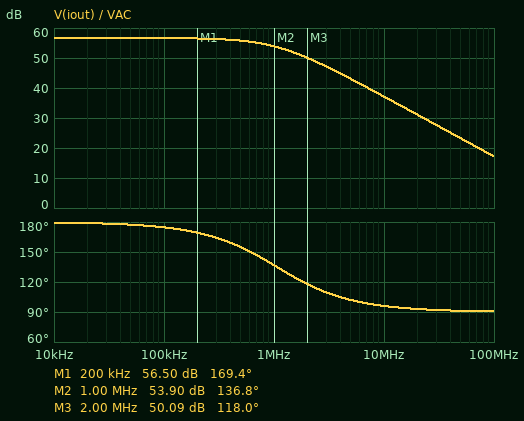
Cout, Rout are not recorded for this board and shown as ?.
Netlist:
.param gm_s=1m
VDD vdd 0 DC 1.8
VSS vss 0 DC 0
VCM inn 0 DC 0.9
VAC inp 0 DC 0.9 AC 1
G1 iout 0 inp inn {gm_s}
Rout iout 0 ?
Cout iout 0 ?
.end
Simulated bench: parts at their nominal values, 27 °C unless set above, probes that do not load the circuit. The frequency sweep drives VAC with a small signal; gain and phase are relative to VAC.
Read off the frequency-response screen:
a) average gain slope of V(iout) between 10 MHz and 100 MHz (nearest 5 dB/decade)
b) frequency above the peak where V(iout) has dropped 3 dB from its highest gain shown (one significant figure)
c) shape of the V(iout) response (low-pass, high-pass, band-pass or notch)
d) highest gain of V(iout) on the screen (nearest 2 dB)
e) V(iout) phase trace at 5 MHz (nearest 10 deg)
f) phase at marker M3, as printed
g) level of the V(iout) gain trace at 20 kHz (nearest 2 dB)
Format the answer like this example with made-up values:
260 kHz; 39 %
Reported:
-20 dB/decade; 1 MHz; low-pass; 56 dB; 100 deg; 118.0 deg; 56 dB
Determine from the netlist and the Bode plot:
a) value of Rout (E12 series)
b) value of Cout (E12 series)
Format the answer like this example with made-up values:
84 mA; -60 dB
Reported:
680 kΩ; 220 fF
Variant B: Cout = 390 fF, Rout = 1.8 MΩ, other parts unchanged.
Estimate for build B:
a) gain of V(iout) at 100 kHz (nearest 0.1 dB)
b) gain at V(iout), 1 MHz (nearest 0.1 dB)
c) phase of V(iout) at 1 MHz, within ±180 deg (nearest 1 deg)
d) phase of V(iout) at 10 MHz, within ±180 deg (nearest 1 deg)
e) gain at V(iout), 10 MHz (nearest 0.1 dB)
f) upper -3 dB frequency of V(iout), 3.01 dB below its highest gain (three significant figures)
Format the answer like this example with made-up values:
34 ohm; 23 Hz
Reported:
64.3 dB; 52.0 dB; 103 deg; 91 deg; 32.2 dB; 227 kHz
